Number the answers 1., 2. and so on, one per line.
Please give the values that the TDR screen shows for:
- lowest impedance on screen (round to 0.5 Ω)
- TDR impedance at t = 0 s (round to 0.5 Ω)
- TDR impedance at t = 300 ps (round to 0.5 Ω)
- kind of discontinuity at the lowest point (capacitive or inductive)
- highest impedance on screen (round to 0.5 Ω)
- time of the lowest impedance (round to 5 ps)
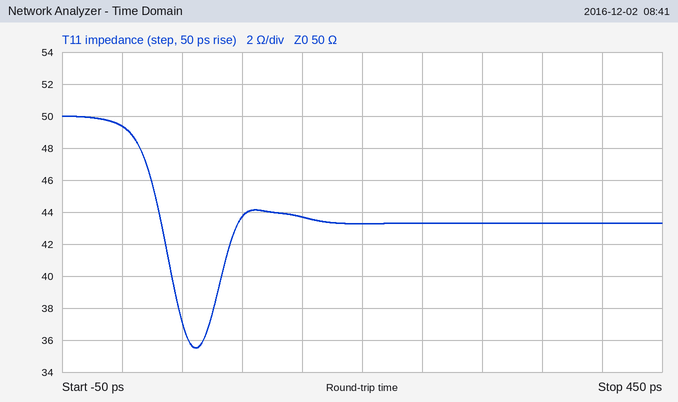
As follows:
1. 35.5 Ω
2. 49.5 Ω
3. 43.5 Ω
4. capacitive
5. 50.0 Ω
6. 60 ps
